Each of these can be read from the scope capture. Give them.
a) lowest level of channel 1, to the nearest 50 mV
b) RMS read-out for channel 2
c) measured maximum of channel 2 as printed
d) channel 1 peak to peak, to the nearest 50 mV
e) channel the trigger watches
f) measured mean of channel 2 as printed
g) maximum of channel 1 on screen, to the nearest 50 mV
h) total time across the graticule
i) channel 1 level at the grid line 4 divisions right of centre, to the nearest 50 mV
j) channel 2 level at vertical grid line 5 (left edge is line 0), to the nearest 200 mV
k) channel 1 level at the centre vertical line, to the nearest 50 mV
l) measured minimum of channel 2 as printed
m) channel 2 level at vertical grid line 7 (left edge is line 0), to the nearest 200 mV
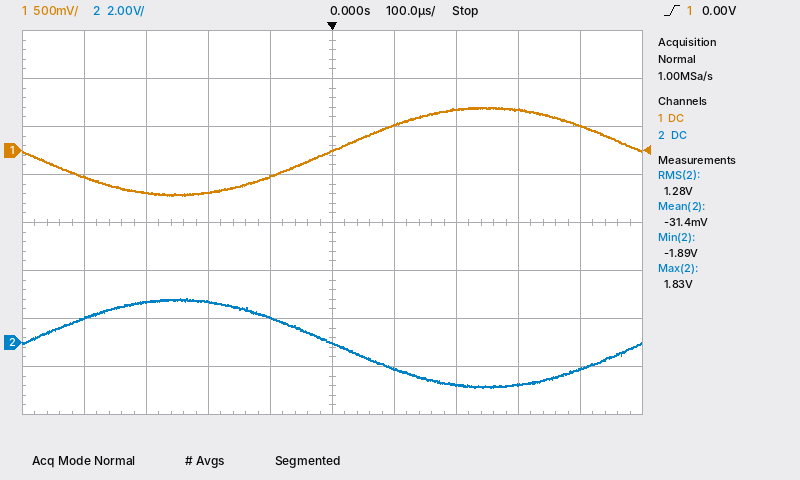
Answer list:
-450 mV
1.28 V
1.83 V
900 mV
channel 1
-31.4 mV
450 mV
1 ms
250 mV
0.0 V
0 mV
-1.89 V
-1.8 V
